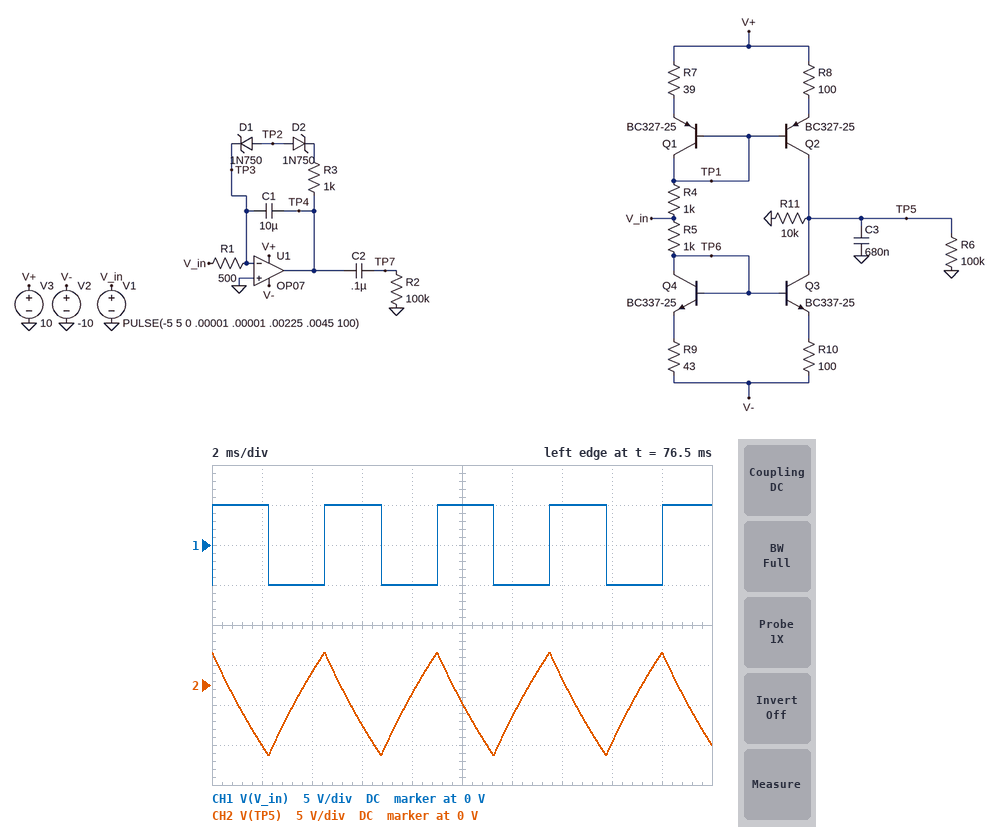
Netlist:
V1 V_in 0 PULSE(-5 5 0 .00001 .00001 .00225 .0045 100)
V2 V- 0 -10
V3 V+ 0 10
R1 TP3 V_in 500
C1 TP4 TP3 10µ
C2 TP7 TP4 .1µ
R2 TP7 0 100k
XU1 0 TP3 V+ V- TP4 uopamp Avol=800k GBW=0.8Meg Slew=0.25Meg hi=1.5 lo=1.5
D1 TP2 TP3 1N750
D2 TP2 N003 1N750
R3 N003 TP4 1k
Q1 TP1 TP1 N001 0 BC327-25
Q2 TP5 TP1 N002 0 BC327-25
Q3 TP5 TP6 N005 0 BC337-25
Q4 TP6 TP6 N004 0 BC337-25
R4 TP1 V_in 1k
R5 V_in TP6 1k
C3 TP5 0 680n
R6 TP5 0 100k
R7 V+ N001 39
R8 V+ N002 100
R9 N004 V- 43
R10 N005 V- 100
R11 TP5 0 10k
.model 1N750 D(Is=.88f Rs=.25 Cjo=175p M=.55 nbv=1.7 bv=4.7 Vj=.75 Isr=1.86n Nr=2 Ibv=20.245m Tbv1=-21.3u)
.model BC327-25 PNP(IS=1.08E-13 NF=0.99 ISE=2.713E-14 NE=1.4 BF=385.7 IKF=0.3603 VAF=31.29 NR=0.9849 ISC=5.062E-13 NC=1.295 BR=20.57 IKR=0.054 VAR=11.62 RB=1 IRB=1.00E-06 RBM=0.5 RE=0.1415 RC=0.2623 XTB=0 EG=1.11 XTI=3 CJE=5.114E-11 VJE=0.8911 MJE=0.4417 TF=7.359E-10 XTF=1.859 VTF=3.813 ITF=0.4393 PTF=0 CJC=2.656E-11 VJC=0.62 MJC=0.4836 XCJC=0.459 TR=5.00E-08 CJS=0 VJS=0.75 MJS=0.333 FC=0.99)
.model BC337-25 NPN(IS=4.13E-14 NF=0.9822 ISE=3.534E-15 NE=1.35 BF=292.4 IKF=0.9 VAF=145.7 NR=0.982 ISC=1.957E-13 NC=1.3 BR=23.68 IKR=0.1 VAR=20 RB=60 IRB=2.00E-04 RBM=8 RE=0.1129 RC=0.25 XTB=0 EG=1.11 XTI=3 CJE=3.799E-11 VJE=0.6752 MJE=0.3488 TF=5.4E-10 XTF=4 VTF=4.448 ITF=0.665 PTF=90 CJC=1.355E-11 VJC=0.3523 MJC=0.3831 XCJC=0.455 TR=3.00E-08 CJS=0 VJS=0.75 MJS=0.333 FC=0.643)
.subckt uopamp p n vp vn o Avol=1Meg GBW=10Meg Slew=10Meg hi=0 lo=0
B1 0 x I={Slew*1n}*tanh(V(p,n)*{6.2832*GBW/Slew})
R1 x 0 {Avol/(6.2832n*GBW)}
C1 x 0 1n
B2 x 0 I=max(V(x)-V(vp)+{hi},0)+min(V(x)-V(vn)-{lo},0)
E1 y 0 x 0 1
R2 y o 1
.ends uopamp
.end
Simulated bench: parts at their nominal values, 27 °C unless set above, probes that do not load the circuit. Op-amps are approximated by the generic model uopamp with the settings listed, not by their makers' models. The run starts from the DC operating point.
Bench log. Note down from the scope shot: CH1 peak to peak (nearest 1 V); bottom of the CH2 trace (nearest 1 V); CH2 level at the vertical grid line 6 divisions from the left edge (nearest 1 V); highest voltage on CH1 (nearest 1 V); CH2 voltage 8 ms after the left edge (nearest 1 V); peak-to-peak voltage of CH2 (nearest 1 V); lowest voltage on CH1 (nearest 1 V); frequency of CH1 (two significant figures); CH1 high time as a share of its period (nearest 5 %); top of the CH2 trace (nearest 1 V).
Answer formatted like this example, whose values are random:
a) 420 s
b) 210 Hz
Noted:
a) 10 V
b) -9 V
c) -4 V
d) 5 V
e) -1 V
f) 13 V
g) -5 V
h) 220 Hz
i) 50 %
j) 4 V
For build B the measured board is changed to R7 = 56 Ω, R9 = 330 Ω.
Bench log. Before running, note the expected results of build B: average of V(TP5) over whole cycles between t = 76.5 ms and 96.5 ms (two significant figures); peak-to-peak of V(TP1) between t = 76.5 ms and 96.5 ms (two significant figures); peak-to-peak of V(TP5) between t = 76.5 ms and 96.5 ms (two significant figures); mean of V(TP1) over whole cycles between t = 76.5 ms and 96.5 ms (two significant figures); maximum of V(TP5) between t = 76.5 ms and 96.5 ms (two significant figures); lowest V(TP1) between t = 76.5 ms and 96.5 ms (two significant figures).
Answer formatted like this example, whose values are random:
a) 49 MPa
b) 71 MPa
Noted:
a) -8.9 V
b) 560 mV
c) 270 mV
d) 8.9 V
e) -8.8 V
f) 8.6 V
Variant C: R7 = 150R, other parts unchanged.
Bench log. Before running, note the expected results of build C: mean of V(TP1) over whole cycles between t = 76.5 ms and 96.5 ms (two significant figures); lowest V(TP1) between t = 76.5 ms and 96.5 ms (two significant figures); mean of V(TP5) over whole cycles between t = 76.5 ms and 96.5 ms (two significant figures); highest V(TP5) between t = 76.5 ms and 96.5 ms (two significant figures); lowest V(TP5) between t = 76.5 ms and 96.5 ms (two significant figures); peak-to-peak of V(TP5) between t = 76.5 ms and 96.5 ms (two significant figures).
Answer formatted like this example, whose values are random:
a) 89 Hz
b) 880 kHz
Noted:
a) 8.5 V
b) 7.5 V
c) 7.8 V
d) 9.1 V
e) 4.8 V
f) 4.3 V
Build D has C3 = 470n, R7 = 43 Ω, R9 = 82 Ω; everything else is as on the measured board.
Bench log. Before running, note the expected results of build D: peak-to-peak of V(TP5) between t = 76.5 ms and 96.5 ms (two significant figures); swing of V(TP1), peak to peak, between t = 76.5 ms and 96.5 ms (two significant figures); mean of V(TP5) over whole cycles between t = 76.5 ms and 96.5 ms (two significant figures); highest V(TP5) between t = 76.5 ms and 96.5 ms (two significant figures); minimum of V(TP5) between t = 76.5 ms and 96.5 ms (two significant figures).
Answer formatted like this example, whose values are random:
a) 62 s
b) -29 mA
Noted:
a) 14 V
b) 440 mV
c) -4.2 V
d) 5.0 V
e) -9.3 V
